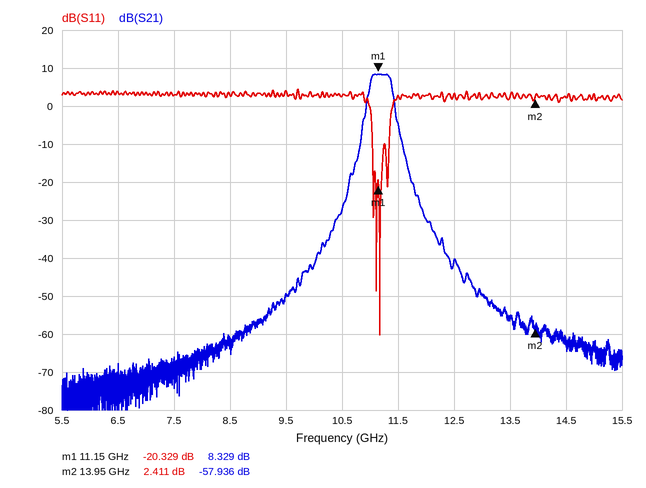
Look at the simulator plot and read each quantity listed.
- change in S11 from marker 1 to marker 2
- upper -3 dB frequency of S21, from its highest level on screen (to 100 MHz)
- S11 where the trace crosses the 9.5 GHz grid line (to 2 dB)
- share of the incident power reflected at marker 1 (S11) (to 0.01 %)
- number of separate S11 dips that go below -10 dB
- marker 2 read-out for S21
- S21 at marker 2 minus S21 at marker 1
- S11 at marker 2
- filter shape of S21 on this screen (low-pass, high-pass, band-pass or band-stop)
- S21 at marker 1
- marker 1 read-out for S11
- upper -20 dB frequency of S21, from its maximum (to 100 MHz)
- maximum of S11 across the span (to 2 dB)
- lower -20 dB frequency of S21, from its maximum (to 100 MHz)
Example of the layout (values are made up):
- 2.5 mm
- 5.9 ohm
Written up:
- 22.740 dB
- 11.4 GHz
- 4 dB
- 0.93 %
- 4
- -57.936 dB
- -66.265 dB
- 2.411 dB
- band-pass
- 8.329 dB
- -20.329 dB
- 11.6 GHz
- 4 dB
- 10.8 GHz
